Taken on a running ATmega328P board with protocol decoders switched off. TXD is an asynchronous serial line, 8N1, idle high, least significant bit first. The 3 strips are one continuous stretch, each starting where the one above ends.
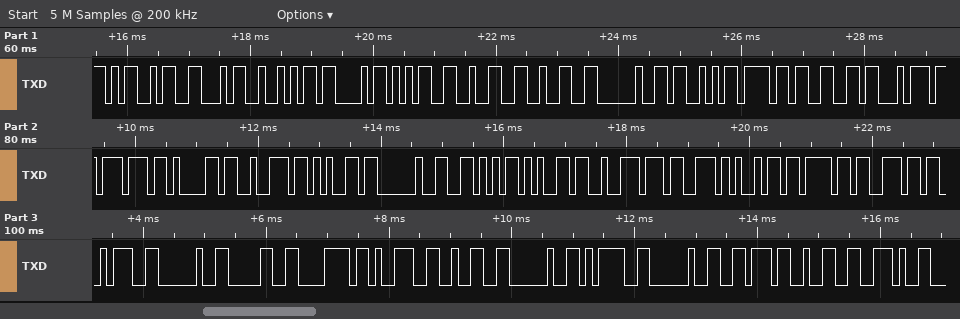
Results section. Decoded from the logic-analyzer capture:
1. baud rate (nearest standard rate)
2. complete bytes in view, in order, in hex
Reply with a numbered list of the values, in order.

1. 9600 baud
2. 4D 46 52 43 35 32 32 20 53 6F 66 74 77 61 72 65 20 56 65 72 73 69 6F 6E 3A 20 30 78 39 32 20 3D 20 76 32 2E
